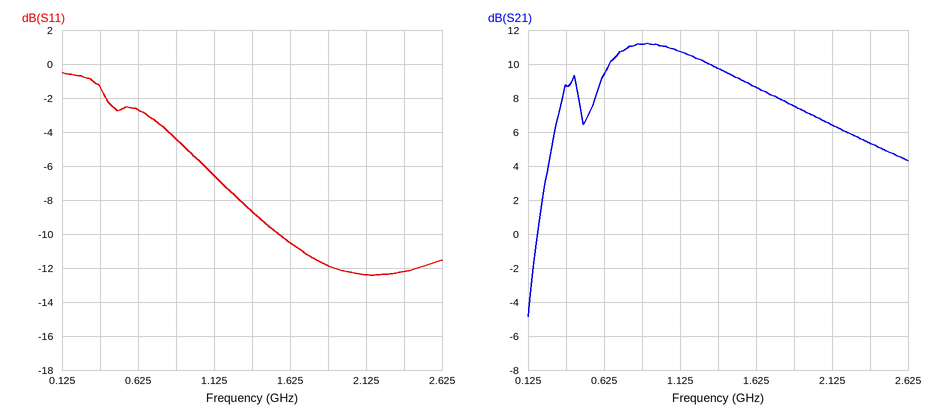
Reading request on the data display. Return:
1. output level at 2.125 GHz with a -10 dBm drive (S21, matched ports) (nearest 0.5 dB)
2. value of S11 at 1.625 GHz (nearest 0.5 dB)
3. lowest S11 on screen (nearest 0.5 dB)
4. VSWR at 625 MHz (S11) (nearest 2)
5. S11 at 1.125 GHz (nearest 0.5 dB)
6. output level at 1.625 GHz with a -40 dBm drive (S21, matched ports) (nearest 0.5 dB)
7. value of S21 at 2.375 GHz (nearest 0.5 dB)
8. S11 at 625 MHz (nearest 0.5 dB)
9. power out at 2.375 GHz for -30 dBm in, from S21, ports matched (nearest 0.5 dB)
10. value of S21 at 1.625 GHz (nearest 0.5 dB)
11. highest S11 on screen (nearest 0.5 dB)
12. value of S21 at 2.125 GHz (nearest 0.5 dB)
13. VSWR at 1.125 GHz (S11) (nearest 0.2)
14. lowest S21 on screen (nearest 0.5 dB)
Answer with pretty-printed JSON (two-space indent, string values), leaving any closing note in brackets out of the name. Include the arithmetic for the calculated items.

{
  "output level at 2.125 GHz with a -10 dBm drive (S21, matched ports)": "-10 dBm + (6.5 dB) = -3.5 dBm",
  "value of S11 at 1.625 GHz": "-10.5 dB",
  "lowest S11 on screen": "-12.5 dB",
  "VSWR at 625 MHz (S11)": "|Γ| = 10^(-2.5/20) = 0.7499; VSWR = (1 + 0.7499)/(1 − 0.7499) ≈ 7.00, so 6 to the nearest 2",
  "S11 at 1.125 GHz": "-6.5 dB",
  "output level at 1.625 GHz with a -40 dBm drive (S21, matched ports)": "-40 dBm + (8.5 dB) = -31.5 dBm",
  "value of S21 at 2.375 GHz": "5.5 dB",
  "S11 at 625 MHz": "-2.5 dB",
  "power out at 2.375 GHz for -30 dBm in, from S21, ports matched": "-30 dBm + (5.5 dB) = -24.5 dBm",
  "value of S21 at 1.625 GHz": "8.5 dB",
  "highest S11 on screen": "-0.5 dB",
  "value of S21 at 2.125 GHz": "6.5 dB",
  "VSWR at 1.125 GHz (S11)": "|Γ| = 10^(-6.5/20) = 0.4732; VSWR = (1 + 0.4732)/(1 − 0.4732) ≈ 2.8",
  "lowest S21 on screen": "-5.0 dB"
}
